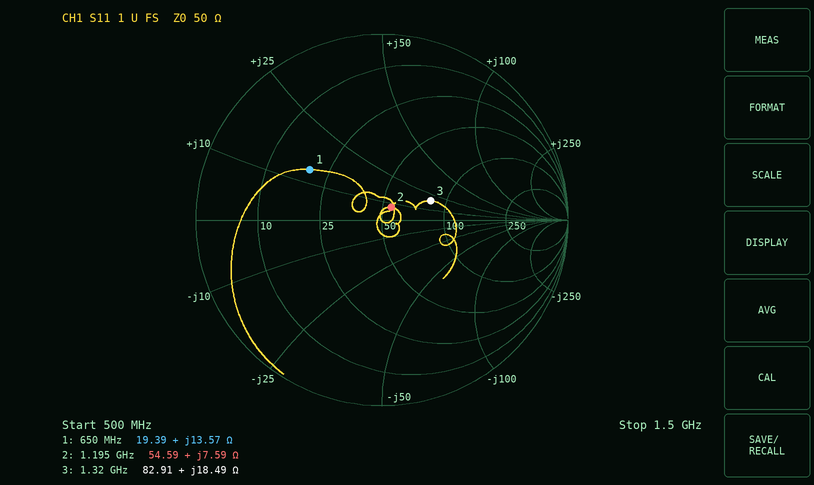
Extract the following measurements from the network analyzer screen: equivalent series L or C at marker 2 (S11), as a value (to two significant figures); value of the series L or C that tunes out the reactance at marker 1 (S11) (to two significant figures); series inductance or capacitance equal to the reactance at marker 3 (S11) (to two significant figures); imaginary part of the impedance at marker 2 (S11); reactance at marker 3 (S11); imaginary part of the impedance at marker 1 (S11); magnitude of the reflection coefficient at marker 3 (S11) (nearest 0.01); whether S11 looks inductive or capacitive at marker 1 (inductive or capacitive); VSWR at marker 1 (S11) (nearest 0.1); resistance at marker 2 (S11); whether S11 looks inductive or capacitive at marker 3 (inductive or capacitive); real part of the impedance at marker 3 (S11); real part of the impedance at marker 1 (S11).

1.0 nH
18 pF
2.2 nH
+7.59 Ω
+18.49 Ω
+13.57 Ω
0.28
inductive
2.8
54.59 Ω
inductive
82.91 Ω
19.39 Ω
